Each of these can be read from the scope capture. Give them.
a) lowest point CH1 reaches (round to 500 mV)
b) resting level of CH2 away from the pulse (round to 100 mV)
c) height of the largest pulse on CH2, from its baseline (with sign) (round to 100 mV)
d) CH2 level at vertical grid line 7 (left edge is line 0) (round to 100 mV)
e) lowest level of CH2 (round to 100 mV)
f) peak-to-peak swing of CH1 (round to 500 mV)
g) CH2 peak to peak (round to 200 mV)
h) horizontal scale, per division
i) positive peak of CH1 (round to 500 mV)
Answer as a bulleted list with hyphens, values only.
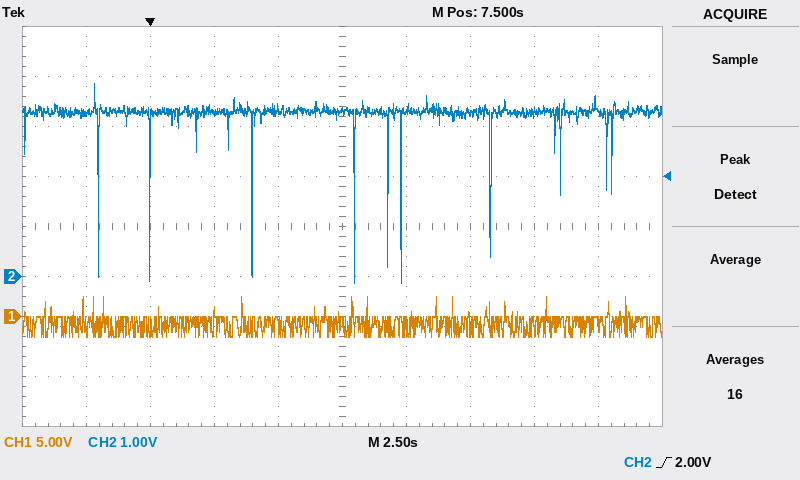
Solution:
- -2.0 V
- 3.3 V
- -3.4 V
- 3.3 V
- -100 mV
- 4.0 V
- 4.0 V
- 2.5 s
- 2.0 V
